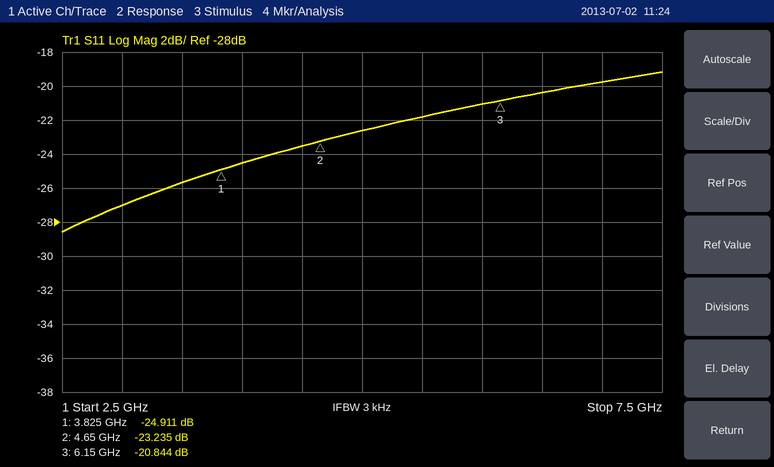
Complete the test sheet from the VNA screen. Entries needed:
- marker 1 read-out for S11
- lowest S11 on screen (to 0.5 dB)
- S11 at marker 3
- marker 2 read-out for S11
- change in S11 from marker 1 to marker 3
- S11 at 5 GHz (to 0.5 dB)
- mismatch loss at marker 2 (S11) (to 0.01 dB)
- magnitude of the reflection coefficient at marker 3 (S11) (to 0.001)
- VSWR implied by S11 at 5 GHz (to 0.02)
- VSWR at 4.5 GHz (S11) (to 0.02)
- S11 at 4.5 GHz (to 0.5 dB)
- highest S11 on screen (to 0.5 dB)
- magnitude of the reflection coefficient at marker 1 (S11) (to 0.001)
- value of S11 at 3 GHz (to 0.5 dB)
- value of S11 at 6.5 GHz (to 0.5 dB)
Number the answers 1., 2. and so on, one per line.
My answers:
1. -24.911 dB
2. -28.5 dB
3. -20.844 dB
4. -23.235 dB
5. 4.067 dB
6. -22.5 dB
7. 0.02 dB
8. 0.091
9. 1.16
10. 1.14
11. -23.5 dB
12. -19.0 dB
13. 0.057
14. -27.0 dB
15. -20.5 dB
